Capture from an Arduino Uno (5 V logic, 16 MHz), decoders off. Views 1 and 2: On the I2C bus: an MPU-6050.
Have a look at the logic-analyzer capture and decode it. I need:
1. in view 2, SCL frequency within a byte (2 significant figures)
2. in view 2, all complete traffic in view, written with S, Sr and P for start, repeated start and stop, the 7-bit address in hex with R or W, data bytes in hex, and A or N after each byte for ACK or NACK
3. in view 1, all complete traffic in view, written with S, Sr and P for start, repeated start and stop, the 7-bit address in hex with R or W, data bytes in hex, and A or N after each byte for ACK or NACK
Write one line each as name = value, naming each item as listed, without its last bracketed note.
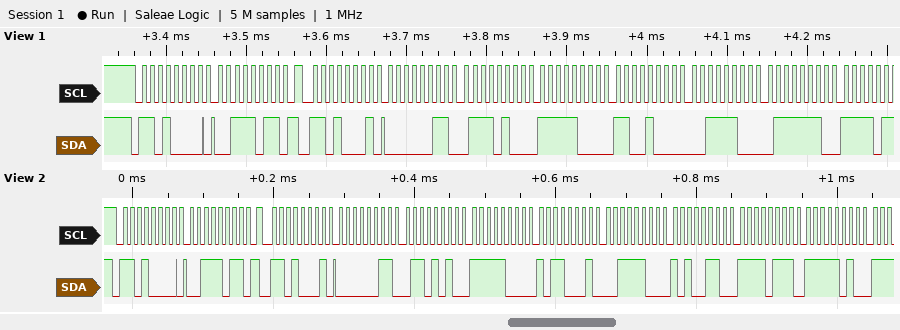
in view 2, SCL frequency within a byte = 100 kHz
in view 2, all complete traffic in view, written with S, Sr and P for start, repeated start and stop, the 7-bit address in hex with R or W, data bytes in hex, and A or N after each byte for ACK or NACK = S 68W A 3B A Sr 68R A 03 A 6A A F8 A B1 A 3C A A6 A F7 A FA A
in view 1, all complete traffic in view, written with S, Sr and P for start, repeated start and stop, the 7-bit address in hex with R or W, data bytes in hex, and A or N after each byte for ACK or NACK = S 68W A 3B A Sr 68R A 03 A 74 A F8 A C8 A 3C A 7E A
